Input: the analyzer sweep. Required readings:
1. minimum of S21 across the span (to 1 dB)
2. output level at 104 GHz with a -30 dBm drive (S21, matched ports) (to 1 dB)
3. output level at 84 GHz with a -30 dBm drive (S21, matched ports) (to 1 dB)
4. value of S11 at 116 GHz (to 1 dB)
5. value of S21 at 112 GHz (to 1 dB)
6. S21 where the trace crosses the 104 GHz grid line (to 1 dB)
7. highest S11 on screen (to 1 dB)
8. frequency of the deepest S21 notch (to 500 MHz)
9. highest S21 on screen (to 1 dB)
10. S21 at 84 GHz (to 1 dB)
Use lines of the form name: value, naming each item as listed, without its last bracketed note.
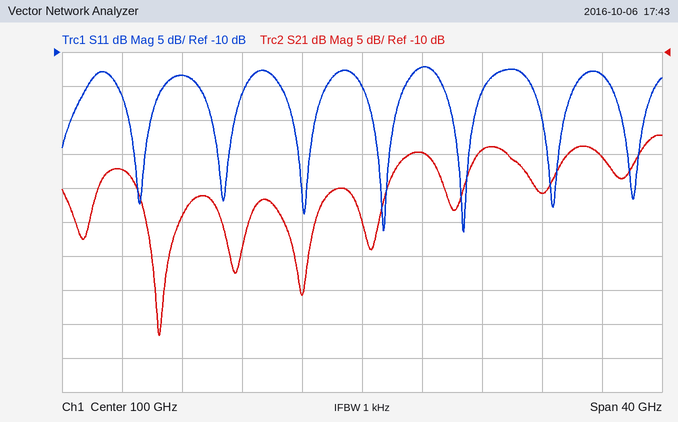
minimum of S21 across the span: -52 dB
output level at 104 GHz with a -30 dBm drive (S21, matched ports): -55 dBm
output level at 84 GHz with a -30 dBm drive (S21, matched ports): -57 dBm
value of S11 at 116 GHz: -13 dB
value of S21 at 112 GHz: -31 dB
S21 where the trace crosses the 104 GHz grid line: -25 dB
highest S11 on screen: -12 dB
frequency of the deepest S21 notch: 86.5 GHz
highest S21 on screen: -22 dB
S21 at 84 GHz: -27 dB
